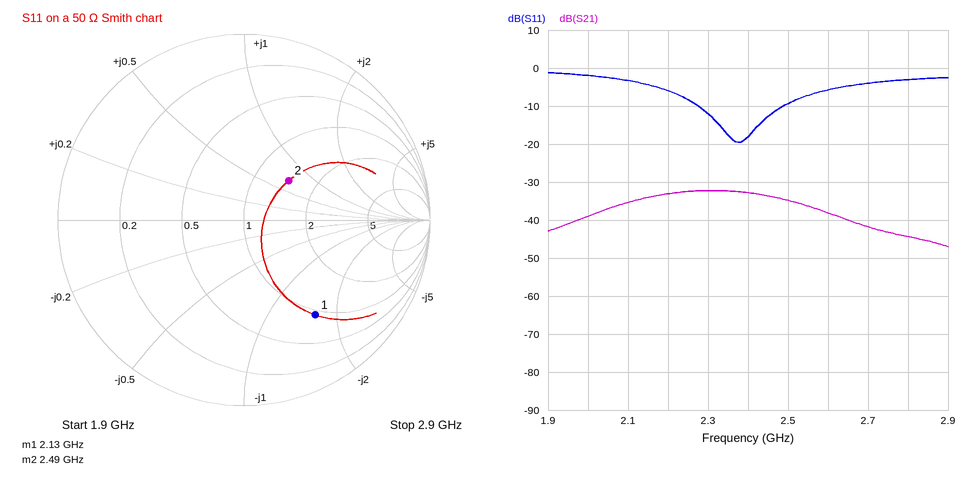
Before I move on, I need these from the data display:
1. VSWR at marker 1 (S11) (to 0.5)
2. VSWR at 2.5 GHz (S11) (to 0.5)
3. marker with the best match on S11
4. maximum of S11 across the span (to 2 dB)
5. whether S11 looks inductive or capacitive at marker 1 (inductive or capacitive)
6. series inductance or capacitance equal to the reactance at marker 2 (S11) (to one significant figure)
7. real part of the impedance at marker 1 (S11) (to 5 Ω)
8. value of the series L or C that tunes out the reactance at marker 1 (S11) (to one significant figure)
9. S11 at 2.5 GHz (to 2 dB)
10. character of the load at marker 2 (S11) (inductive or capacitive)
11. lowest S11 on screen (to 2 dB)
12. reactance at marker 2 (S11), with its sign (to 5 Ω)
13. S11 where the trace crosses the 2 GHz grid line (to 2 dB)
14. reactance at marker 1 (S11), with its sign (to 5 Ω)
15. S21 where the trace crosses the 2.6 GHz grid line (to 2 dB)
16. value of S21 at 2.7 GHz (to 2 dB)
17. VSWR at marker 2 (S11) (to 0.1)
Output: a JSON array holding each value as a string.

["4.5", "2.0", "marker 2", "-2 dB", "capacitive", "2 nH", "45 Ω", "6 nH", "-10 dB", "inductive", "-20 dB", "+35 Ω", "-2 dB", "-80 Ω", "-38 dB", "-42 dB", "1.9"]
